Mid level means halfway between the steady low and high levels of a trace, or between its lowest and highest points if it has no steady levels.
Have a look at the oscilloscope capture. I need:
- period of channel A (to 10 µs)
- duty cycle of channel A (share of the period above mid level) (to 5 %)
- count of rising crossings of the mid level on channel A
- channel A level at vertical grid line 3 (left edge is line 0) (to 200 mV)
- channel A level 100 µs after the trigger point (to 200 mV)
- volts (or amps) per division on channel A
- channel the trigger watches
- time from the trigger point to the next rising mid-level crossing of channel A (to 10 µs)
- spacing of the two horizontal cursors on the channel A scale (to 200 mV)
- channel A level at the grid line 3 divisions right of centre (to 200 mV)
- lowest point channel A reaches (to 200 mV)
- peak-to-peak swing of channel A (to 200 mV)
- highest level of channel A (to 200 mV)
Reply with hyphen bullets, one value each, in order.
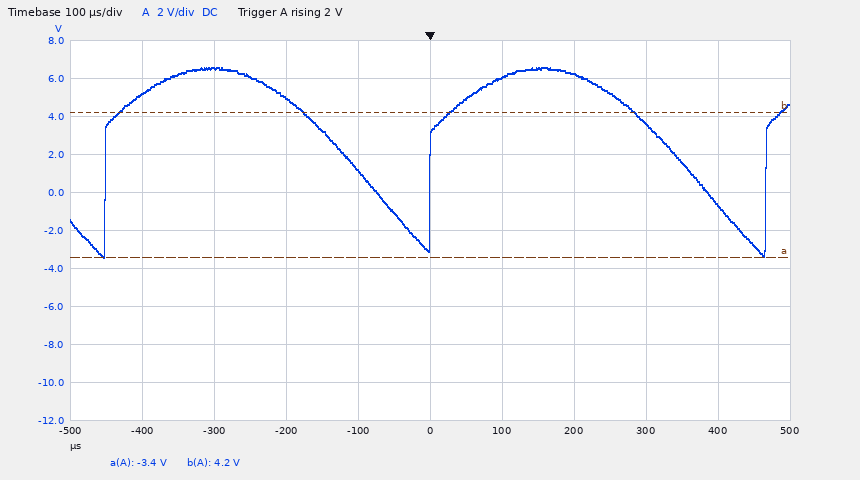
- 460 µs
- 75 %
- 3
- 5.0 V
- 6.0 V
- 2 V
- channel A
- 470 µs
- 7.6 V
- 3.6 V
- -3.4 V
- 10.0 V
- 6.6 V
